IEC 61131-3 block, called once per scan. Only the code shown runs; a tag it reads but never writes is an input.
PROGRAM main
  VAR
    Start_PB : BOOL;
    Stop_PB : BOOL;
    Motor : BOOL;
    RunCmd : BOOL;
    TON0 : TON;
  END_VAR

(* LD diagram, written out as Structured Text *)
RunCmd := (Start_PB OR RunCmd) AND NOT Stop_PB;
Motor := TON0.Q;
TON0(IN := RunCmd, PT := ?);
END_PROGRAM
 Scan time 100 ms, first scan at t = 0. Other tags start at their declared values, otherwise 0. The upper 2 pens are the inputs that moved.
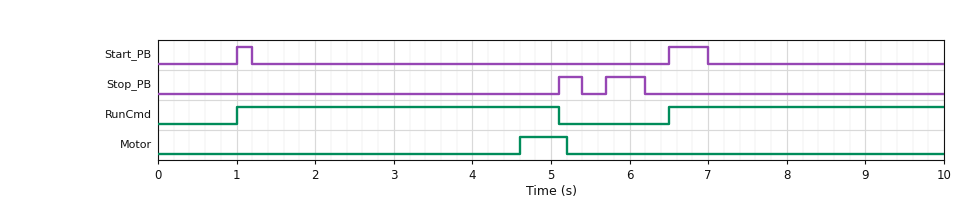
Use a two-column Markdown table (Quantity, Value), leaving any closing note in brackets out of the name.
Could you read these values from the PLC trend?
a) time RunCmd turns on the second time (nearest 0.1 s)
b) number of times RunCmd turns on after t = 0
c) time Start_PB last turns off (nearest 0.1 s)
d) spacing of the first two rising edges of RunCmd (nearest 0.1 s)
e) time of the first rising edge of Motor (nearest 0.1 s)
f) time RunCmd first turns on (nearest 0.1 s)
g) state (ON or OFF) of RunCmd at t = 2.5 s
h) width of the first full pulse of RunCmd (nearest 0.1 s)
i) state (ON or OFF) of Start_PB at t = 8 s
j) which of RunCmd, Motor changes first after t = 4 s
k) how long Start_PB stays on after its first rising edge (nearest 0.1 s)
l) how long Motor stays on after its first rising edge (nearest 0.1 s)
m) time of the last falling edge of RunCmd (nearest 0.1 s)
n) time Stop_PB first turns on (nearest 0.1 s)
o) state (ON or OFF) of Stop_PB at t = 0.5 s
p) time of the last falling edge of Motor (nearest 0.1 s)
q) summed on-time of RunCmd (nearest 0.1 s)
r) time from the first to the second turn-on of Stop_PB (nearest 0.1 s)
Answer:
| Quantity | Value |
|---|---|
| time RunCmd turns on the second time | 6.5 s |
| number of times RunCmd turns on after t = 0 | 2 |
| time Start_PB last turns off | 7.0 s |
| spacing of the first two rising edges of RunCmd | 5.5 s |
| time of the first rising edge of Motor | 4.6 s |
| time RunCmd first turns on | 1.0 s |
| state (ON or OFF) of RunCmd at t = 2.5 s | ON |
| width of the first full pulse of RunCmd | 4.1 s |
| state (ON or OFF) of Start_PB at t = 8 s | OFF |
| which of RunCmd, Motor changes first after t = 4 s | Motor |
| how long Start_PB stays on after its first rising edge | 0.2 s |
| how long Motor stays on after its first rising edge | 0.6 s |
| time of the last falling edge of RunCmd | 5.1 s |
| time Stop_PB first turns on | 5.1 s |
| state (ON or OFF) of Stop_PB at t = 0.5 s | OFF |
| time of the last falling edge of Motor | 5.2 s |
| summed on-time of RunCmd | 7.6 s |
| time from the first to the second turn-on of Stop_PB | 0.6 s |
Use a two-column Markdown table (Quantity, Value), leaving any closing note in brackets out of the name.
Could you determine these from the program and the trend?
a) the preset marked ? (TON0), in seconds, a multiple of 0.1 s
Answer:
| Quantity | Value |
|---|---|
| the preset marked ? (TON0), in seconds, a multiple of 0.1 s | 3.5 s |
